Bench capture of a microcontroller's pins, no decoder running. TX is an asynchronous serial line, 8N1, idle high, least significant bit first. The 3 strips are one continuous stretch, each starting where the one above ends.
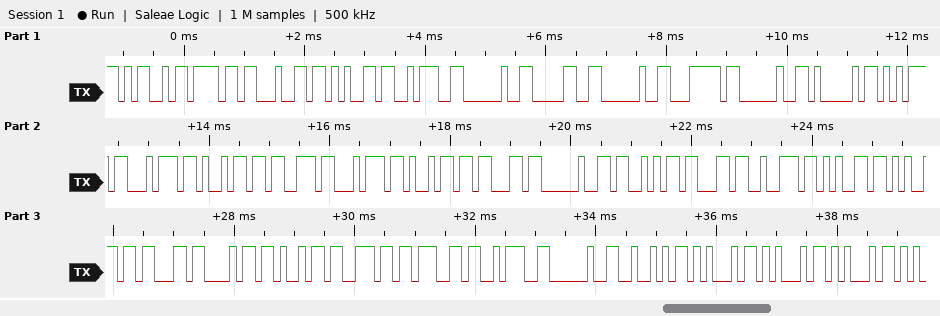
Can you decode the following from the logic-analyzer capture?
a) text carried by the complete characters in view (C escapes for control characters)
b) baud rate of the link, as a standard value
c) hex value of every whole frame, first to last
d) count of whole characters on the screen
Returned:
"Mode: 0 | Autistic Screeching: REEE"
9600 baud
4D 6F 64 65 3A 20 30 20 7C 20 41 75 74 69 73 74 69 63 20 53 63 72 65 65 63 68 69 6E 67 3A 20 52 45 45 45
35
